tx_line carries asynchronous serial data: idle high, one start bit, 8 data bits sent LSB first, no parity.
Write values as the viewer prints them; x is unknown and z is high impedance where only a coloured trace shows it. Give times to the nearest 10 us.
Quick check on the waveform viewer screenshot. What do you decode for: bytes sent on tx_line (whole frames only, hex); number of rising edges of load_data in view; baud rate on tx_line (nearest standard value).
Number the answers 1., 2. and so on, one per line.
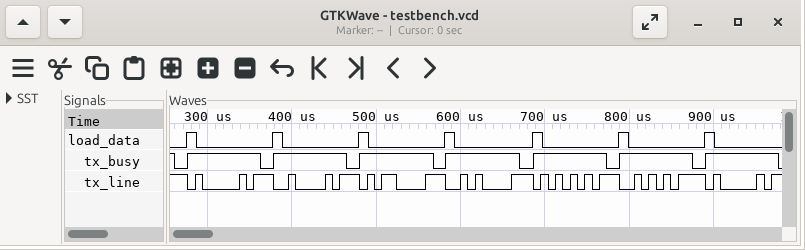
1. 41, 42, 0D, 0A, 55, AA, 41
2. 7
3. 115200 baud
